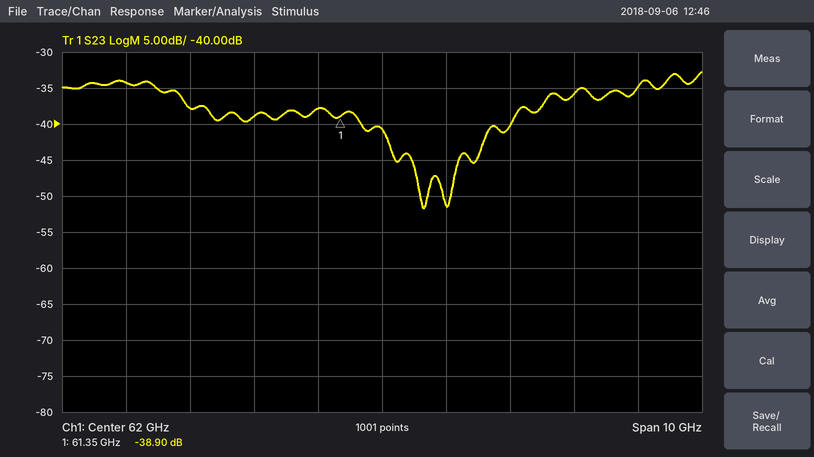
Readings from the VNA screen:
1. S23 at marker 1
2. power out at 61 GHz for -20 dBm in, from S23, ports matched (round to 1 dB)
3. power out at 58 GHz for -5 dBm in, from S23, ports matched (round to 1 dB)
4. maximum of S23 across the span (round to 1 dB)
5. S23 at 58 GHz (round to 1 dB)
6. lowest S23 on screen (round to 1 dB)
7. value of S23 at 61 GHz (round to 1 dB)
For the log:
-38.90 dB
-58 dBm
-39 dBm
-33 dB
-34 dB
-52 dB
-38 dB
